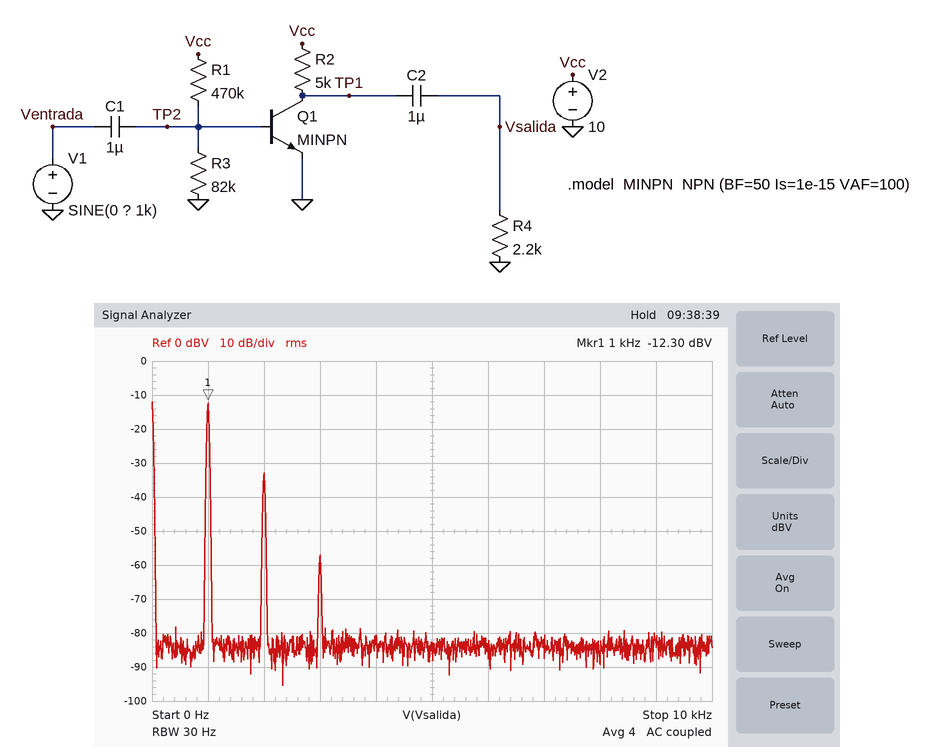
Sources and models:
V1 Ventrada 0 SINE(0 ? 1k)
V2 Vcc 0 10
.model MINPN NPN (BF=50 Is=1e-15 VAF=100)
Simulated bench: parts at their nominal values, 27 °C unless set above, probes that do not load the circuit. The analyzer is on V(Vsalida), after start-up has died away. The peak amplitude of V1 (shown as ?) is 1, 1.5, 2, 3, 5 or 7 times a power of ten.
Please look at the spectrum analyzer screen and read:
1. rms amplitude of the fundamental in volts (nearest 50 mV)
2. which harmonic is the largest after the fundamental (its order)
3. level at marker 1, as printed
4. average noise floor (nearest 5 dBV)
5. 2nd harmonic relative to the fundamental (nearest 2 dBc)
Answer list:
250 mV
2
-12.30 dBV
-85 dBV
-20 dBc
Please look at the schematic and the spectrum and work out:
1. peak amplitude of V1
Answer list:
10 mV
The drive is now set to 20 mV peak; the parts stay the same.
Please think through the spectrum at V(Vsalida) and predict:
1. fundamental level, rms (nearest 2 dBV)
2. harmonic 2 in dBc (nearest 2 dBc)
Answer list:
-6 dBV
-14 dBc
